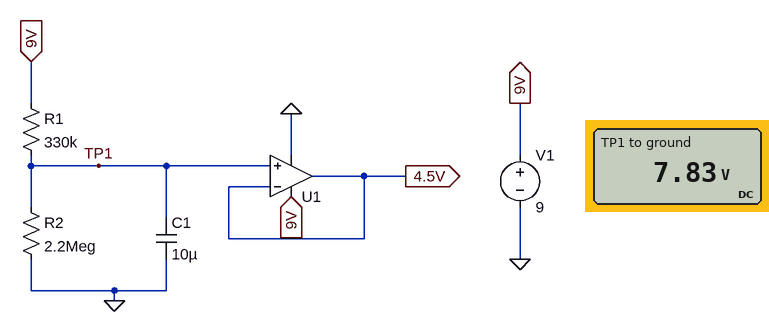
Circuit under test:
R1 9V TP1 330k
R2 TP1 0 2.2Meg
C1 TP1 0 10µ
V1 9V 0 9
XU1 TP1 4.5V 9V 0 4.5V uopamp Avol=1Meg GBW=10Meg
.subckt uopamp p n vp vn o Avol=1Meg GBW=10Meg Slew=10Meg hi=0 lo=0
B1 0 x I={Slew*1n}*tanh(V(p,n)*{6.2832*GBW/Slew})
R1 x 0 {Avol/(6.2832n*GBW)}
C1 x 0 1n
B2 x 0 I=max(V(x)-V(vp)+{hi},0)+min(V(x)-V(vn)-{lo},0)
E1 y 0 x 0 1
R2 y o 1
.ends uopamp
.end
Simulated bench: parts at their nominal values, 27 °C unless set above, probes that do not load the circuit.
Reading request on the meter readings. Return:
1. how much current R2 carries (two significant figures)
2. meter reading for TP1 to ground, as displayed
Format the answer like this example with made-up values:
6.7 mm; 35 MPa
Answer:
3.6 µA; 7.83 V
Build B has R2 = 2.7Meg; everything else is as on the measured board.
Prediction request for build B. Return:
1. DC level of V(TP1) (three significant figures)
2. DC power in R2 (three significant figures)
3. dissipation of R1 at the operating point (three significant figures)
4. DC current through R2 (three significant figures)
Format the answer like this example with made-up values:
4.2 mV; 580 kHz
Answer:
8.02 V; 23.8 µW; 2.91 µW; 2.97 µA
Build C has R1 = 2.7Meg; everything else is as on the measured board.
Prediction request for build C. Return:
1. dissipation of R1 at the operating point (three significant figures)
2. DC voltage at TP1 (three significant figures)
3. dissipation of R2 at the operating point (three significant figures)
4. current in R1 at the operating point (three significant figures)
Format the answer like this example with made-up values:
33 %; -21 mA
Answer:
9.11 µW; 4.04 V; 7.42 µW; 1.84 µA
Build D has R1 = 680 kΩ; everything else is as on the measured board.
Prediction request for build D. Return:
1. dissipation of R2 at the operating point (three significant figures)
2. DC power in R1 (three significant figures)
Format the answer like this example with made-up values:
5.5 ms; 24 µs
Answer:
21.5 µW; 6.64 µW
